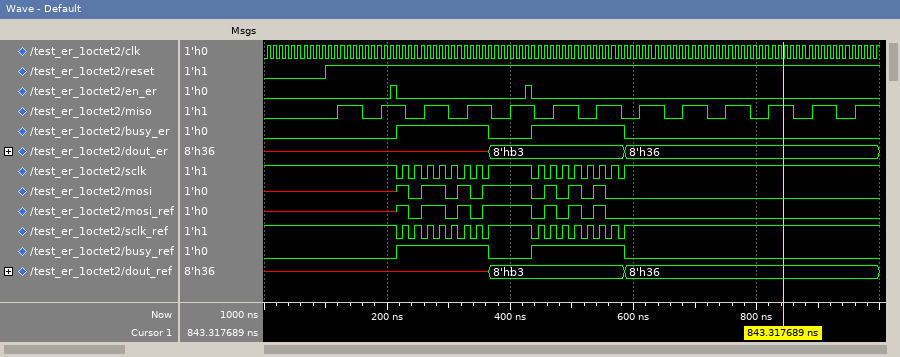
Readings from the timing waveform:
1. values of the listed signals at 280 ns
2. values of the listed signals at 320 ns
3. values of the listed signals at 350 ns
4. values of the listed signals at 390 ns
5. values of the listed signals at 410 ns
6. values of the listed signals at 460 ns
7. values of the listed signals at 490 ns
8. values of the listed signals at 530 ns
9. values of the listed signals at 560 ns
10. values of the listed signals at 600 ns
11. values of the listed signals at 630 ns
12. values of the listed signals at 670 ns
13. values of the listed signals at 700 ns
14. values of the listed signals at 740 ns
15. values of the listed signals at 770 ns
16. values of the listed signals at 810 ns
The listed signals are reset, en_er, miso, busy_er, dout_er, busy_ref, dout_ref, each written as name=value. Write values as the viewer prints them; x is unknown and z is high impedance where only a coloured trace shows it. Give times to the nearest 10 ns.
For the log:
reset=1, en_er=0, miso=1, busy_er=1, dout_er=x, busy_ref=1, dout_ref=x
reset=1, en_er=0, miso=0, busy_er=1, dout_er=x, busy_ref=1, dout_ref=x
reset=1, en_er=0, miso=1, busy_er=1, dout_er=x, busy_ref=1, dout_ref=x
reset=1, en_er=0, miso=0, busy_er=0, dout_er=8'hb3, busy_ref=0, dout_ref=8'hb3
reset=1, en_er=0, miso=1, busy_er=0, dout_er=8'hb3, busy_ref=0, dout_ref=8'hb3
reset=1, en_er=0, miso=0, busy_er=1, dout_er=8'hb3, busy_ref=1, dout_ref=8'hb3
reset=1, en_er=0, miso=1, busy_er=1, dout_er=8'hb3, busy_ref=1, dout_ref=8'hb3
reset=1, en_er=0, miso=0, busy_er=1, dout_er=8'hb3, busy_ref=1, dout_ref=8'hb3
reset=1, en_er=0, miso=1, busy_er=1, dout_er=8'hb3, busy_ref=1, dout_ref=8'hb3
reset=1, en_er=0, miso=0, busy_er=0, dout_er=8'h36, busy_ref=0, dout_ref=8'h36
reset=1, en_er=0, miso=1, busy_er=0, dout_er=8'h36, busy_ref=0, dout_ref=8'h36
reset=1, en_er=0, miso=0, busy_er=0, dout_er=8'h36, busy_ref=0, dout_ref=8'h36
reset=1, en_er=0, miso=1, busy_er=0, dout_er=8'h36, busy_ref=0, dout_ref=8'h36
reset=1, en_er=0, miso=0, busy_er=0, dout_er=8'h36, busy_ref=0, dout_ref=8'h36
reset=1, en_er=0, miso=1, busy_er=0, dout_er=8'h36, busy_ref=0, dout_ref=8'h36
reset=1, en_er=0, miso=0, busy_er=0, dout_er=8'h36, busy_ref=0, dout_ref=8'h36
